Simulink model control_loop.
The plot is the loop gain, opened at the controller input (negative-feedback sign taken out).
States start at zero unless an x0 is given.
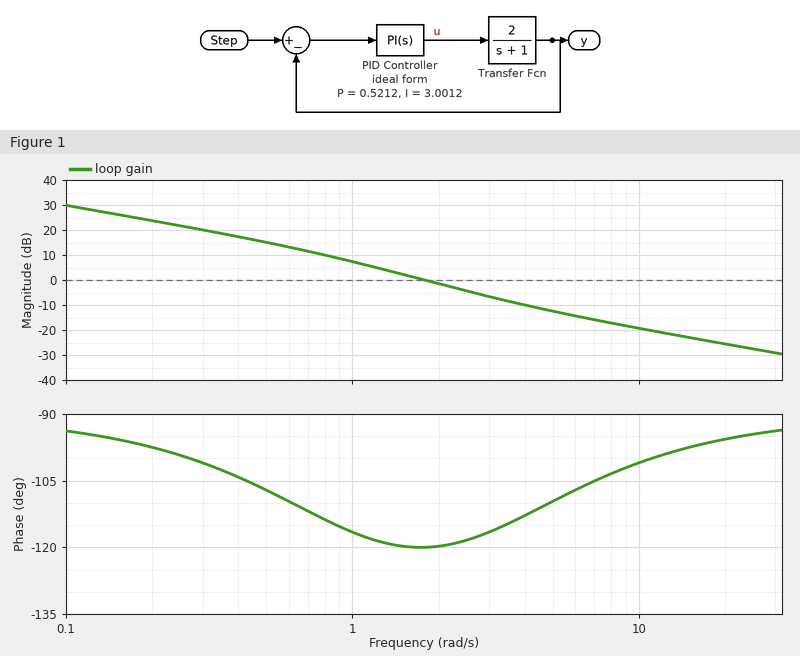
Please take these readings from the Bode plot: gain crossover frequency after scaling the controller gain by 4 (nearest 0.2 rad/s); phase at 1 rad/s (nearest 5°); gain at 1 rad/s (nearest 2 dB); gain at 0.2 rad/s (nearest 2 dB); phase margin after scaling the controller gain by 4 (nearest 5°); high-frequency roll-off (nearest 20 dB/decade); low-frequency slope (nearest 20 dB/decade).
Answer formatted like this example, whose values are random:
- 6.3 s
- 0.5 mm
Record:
- 4.8 rad/s
- -115°
- 8 dB
- 24 dB
- 70°
- -20 dB/decade
- -20 dB/decade
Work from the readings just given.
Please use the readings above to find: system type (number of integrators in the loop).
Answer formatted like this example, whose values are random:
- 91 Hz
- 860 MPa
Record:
- 1
